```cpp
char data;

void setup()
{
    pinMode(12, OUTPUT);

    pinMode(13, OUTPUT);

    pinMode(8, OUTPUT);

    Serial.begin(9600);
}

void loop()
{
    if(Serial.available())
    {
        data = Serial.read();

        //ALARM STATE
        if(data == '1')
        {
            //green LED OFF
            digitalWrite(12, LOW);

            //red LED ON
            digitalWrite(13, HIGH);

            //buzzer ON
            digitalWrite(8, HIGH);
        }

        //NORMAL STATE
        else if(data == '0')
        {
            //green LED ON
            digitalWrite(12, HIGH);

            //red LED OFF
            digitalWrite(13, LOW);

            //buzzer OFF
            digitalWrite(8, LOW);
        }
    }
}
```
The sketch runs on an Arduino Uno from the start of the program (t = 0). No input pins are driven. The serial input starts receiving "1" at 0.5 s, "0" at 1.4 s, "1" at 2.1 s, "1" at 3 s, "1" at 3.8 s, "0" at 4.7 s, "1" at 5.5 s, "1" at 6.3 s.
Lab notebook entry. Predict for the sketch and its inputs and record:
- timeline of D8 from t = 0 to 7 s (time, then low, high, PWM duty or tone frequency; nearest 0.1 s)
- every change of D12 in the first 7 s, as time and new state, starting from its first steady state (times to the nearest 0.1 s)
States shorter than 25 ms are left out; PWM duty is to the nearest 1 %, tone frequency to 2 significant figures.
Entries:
0 s low; 0.5 s high; 1.4 s low; 2.1 s high; 4.7 s low; 5.5 s high
0 s low; 1.4 s high; 2.1 s low; 4.7 s high; 5.5 s low
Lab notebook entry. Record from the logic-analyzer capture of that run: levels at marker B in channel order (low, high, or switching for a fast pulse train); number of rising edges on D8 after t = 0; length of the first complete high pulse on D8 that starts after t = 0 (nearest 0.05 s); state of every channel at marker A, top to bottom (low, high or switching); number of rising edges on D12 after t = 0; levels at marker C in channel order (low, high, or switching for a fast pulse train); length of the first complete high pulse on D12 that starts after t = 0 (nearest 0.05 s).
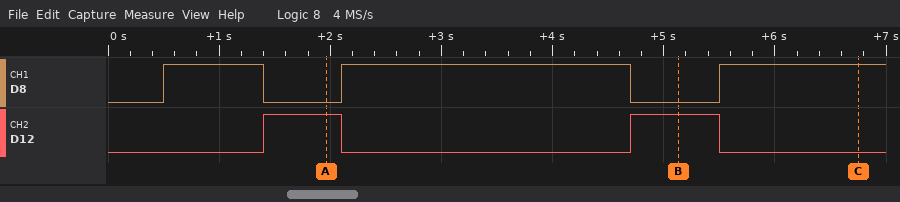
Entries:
D8 low, D12 high
3
0.90 s
D8 low, D12 high
2
D8 high, D12 low
0.70 s
